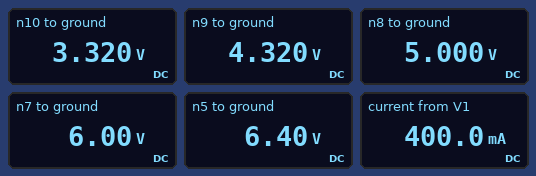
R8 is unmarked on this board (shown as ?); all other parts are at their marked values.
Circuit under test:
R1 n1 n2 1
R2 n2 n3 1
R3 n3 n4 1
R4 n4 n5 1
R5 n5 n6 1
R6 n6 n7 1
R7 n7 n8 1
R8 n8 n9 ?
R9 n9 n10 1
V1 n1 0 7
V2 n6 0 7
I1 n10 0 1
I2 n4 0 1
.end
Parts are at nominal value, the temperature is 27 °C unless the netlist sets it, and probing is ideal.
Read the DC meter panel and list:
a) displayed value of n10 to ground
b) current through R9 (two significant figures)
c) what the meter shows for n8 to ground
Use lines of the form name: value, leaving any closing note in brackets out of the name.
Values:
displayed value of n10 to ground: 3.320 V
current through R9: 1.0 A
what the meter shows for n8 to ground: 5.000 V
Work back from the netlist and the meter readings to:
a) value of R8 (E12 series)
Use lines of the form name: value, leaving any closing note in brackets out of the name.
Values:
value of R8: 0.68 Ω
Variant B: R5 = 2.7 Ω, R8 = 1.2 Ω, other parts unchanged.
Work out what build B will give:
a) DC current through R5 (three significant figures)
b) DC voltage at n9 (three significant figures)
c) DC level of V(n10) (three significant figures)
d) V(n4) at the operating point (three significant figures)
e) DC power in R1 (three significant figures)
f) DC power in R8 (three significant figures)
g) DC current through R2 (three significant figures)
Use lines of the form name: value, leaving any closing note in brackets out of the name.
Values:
DC current through R5: 448 mA
DC voltage at n9: 3.80 V
DC level of V(n10): 2.80 V
V(n4) at the operating point: 5.34 V
DC power in R1: 305 mW
DC power in R8: 1.20 W
DC current through R2: 552 mA
